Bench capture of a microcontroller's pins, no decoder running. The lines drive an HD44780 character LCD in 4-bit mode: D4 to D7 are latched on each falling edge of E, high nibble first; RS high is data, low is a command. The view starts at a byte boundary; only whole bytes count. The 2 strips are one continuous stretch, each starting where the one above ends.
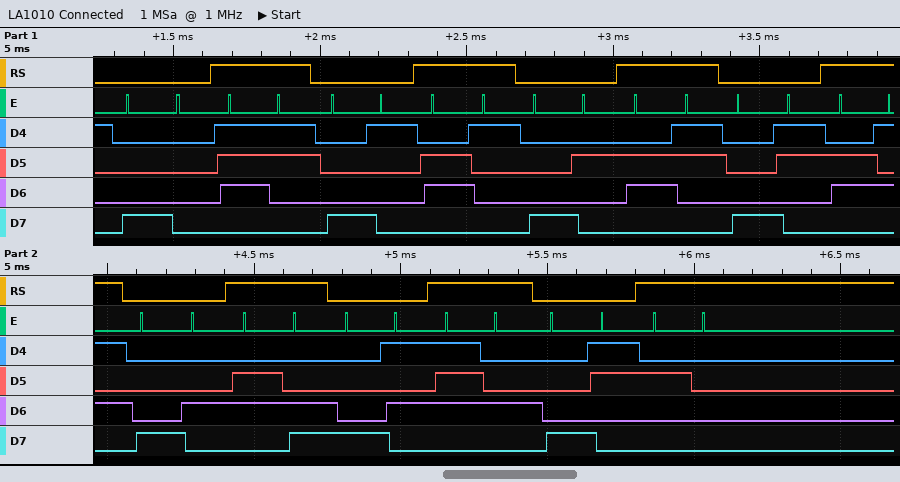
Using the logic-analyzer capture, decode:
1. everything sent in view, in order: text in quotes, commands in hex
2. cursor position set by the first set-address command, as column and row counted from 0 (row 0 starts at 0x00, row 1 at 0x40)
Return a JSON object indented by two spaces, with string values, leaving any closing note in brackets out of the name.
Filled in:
{
  "everything sent in view, in order: text in quotes, commands in hex": "0x80 \"s\" 0x81 \"a\" 0x82 \"c\" 0x83 \"e\" 0x84 \"l\" 0x85 \"t\" 0x83 \" \"",
  "cursor position set by the first set-address command, as column and row counted from 0": "column 0, row 0"
}
